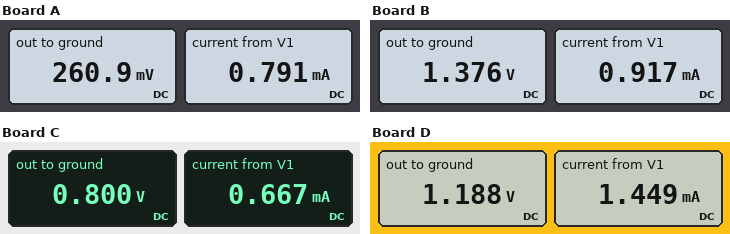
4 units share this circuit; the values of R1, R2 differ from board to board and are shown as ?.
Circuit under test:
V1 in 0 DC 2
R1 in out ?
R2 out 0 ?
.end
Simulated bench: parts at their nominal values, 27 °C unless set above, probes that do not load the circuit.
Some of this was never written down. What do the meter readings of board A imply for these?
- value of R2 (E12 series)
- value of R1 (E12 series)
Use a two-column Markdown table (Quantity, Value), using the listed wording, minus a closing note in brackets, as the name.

| Quantity | Value |
|---|---|
| value of R2 | 330 Ω |
| value of R1 | 2.2 kΩ |
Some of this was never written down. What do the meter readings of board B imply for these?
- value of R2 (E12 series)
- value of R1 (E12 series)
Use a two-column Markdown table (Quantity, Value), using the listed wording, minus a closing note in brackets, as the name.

| Quantity | Value |
|---|---|
| value of R2 | 1.5 kΩ |
| value of R1 | 680 Ω |
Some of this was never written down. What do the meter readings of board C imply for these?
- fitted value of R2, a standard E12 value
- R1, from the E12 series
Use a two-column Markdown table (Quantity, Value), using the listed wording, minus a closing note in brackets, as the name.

| Quantity | Value |
|---|---|
| fitted value of R2, a standard E12 value | 1.2 kΩ |
| R1, from the E12 series | 1.8 kΩ |
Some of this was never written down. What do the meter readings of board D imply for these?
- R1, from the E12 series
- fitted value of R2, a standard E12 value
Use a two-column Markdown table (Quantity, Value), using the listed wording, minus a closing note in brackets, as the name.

| Quantity | Value |
|---|---|
| R1, from the E12 series | 560 Ω |
| fitted value of R2, a standard E12 value | 820 Ω |
